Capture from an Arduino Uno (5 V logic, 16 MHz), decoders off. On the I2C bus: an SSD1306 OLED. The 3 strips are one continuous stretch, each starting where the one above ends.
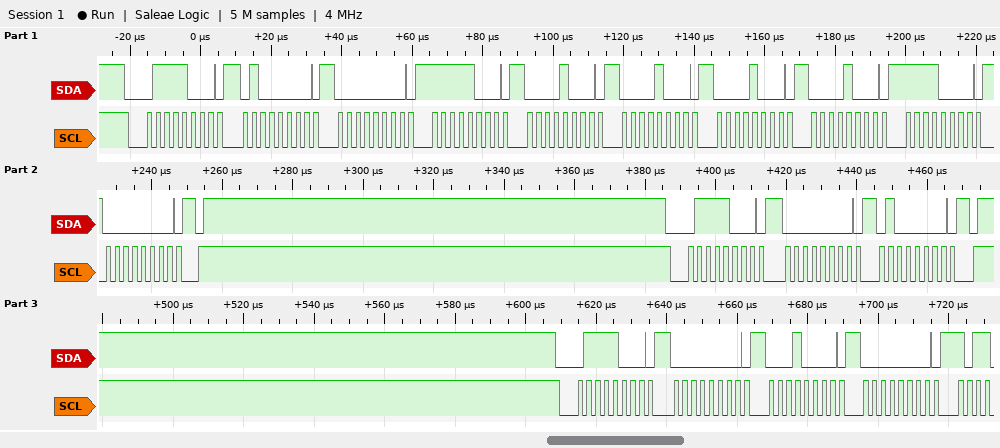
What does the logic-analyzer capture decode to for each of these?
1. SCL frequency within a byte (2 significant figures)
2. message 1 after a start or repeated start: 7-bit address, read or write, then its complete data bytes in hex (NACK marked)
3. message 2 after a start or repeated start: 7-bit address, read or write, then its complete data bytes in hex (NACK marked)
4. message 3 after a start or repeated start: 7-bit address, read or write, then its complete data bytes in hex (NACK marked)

400 kHz
0x3C write: 40 00 F8 08 08 08 08 F0 00
0x3C write: 00 40
0x3C write: 00 10 00
